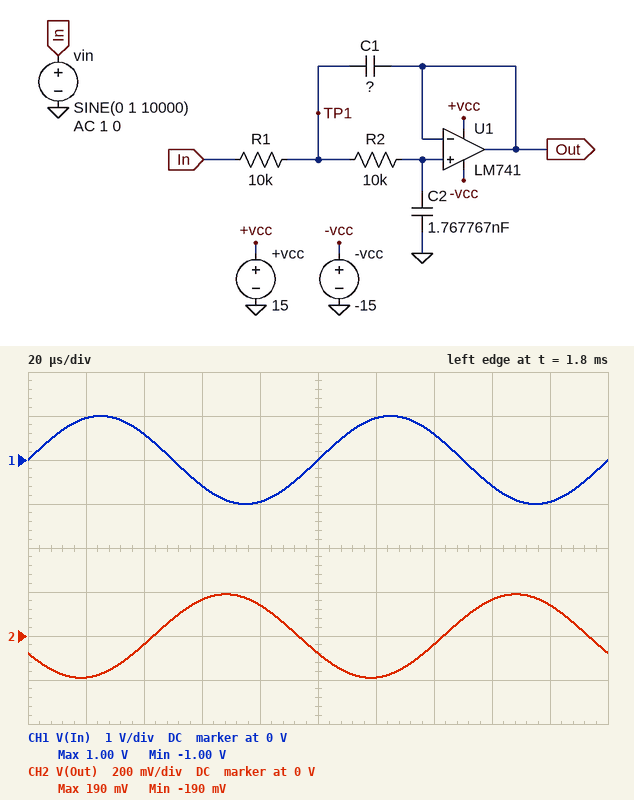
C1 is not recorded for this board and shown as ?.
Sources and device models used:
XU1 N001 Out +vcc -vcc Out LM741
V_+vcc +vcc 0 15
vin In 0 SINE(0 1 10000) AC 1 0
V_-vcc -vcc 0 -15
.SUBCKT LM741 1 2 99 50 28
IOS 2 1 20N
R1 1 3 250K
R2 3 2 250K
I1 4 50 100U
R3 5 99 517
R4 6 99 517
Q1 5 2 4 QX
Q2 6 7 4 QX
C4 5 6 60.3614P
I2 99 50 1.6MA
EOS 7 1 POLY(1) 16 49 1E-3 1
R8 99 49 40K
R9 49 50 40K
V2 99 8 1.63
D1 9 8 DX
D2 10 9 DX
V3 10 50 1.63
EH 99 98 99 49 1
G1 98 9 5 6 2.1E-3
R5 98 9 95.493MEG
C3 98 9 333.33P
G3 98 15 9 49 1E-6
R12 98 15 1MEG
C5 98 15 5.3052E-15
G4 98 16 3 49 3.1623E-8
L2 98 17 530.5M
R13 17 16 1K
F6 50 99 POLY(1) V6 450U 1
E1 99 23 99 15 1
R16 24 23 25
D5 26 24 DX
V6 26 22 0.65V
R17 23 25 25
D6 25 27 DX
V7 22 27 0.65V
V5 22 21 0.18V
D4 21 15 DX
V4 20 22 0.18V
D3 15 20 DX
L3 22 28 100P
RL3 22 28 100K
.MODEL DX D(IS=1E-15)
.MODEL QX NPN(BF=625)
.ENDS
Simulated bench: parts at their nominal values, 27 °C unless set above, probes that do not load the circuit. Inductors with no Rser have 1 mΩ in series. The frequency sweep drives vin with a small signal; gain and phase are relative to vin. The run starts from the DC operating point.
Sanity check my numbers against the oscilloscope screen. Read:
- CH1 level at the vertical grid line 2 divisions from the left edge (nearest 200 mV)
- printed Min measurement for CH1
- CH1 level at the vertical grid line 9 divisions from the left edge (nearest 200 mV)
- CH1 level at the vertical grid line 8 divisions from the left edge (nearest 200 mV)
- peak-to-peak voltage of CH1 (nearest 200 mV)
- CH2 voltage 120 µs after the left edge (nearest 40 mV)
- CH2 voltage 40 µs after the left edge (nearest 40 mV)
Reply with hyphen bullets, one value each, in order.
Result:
- 600 mV
- -1.00 V
- -1.0 V
- -600 mV
- 2.0 V
- -200 mV
- -40 mV
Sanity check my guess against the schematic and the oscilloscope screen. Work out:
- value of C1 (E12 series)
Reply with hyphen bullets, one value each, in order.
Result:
- 8.2 nF
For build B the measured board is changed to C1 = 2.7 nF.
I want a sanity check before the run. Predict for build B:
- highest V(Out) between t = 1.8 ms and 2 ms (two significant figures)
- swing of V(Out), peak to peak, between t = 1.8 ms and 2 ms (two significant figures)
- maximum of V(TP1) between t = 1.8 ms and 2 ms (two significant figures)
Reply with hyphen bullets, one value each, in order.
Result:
- 420 mV
- 830 mV
- 620 mV
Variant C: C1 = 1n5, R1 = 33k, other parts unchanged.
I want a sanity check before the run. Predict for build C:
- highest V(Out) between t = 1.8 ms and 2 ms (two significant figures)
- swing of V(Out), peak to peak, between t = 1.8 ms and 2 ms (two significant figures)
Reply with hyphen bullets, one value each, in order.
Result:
- 180 mV
- 370 mV
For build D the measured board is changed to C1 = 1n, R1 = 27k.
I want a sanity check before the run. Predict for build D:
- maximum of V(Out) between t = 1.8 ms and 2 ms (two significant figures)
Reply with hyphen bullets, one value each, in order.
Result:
- 240 mV
